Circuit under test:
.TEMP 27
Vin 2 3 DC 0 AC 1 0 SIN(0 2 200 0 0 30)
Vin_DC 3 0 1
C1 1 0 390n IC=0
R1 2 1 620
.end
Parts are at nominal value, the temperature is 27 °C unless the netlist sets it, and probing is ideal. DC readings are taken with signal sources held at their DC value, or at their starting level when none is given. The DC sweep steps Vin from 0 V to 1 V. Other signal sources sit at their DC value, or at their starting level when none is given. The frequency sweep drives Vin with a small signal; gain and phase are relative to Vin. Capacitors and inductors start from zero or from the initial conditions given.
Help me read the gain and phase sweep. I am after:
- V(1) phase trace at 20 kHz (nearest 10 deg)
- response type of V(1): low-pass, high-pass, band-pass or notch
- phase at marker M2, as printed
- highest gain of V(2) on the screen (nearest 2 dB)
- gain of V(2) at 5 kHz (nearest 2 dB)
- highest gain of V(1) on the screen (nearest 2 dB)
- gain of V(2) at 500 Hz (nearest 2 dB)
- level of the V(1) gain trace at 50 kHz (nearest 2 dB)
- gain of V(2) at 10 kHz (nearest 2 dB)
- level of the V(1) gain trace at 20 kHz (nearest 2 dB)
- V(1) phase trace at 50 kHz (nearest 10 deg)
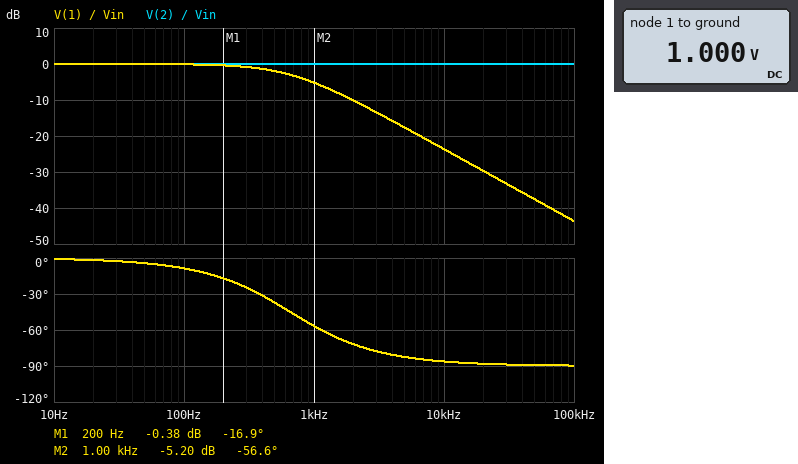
-90 deg
low-pass
-56.6 deg
0 dB
0 dB
0 dB
0 dB
-38 dB
0 dB
-30 dB
-90 deg
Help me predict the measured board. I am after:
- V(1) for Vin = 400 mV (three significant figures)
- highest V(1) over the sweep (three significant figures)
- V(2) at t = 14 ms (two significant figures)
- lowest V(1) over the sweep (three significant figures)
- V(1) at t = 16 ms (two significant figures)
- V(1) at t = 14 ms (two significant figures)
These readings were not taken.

1.40 V
2.00 V
-340 mV
1.00 V
2.9 V
-640 mV
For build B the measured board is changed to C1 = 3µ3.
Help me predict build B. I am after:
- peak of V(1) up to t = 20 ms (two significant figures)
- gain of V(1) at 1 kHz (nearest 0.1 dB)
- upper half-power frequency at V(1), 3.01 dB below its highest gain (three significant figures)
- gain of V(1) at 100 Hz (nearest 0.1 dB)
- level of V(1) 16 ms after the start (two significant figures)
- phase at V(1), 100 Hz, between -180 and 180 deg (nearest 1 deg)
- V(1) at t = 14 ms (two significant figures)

1.7 V
-22.2 dB
77.8 Hz
-4.2 dB
1.4 V
-52 deg
320 mV
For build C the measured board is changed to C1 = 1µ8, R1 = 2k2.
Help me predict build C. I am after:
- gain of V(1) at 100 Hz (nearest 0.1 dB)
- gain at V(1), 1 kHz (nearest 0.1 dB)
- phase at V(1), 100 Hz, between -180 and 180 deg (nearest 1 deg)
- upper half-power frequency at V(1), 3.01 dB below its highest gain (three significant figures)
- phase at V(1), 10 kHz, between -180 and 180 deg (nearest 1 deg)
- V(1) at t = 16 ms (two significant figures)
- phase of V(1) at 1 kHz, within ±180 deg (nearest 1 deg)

-8.6 dB
-27.9 dB
-68 deg
40.2 Hz
-90 deg
1.1 V
-88 deg
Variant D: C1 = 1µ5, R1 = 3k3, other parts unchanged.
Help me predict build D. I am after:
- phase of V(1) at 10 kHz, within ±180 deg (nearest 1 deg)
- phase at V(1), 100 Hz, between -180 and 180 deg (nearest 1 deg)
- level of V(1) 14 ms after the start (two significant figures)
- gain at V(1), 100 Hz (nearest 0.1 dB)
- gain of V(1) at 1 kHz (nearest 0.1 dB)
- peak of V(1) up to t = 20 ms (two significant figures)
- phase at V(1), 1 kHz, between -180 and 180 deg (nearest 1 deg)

-90 deg
-72 deg
690 mV
-10.3 dB
-29.9 dB
1.3 V
-88 deg
